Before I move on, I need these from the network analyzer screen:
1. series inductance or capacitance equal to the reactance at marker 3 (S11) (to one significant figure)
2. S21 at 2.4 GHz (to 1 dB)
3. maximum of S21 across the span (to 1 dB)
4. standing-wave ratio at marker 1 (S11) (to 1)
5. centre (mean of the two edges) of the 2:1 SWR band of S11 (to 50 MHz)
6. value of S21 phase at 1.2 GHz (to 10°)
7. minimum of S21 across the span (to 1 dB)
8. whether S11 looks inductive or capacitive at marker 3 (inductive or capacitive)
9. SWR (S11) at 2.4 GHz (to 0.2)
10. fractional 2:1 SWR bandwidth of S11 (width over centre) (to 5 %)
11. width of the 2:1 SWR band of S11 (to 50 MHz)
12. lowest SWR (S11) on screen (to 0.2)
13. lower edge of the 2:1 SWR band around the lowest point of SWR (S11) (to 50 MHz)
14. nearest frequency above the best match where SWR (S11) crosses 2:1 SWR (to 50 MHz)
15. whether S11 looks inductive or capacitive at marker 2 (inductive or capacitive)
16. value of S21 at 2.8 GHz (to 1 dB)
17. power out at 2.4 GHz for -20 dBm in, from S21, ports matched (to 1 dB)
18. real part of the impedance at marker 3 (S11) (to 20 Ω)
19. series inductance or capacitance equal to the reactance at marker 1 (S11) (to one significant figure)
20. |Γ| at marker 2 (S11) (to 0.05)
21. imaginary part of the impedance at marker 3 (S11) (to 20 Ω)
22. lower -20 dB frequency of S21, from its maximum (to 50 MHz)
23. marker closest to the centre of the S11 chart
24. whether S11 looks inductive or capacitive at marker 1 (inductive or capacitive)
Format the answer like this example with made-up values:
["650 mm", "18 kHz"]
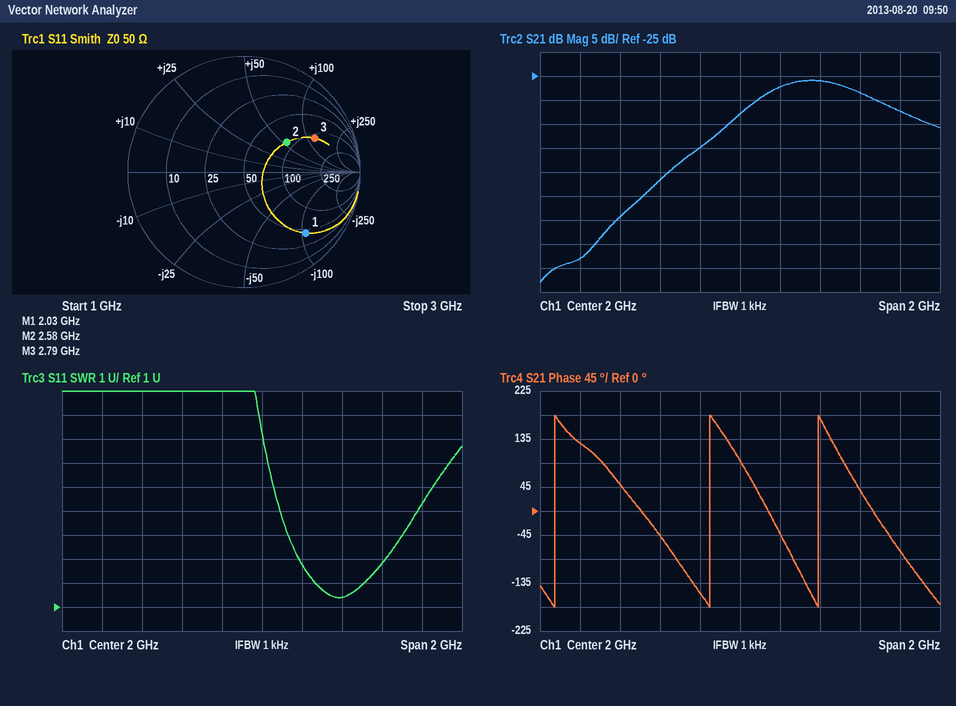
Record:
["7 nH", "-26 dB", "-26 dB", "7", "2.40 GHz", "130°", "-68 dB", "inductive", "1.4", "10 %", "250 MHz", "1.4", "2.25 GHz", "2.50 GHz", "inductive", "-32 dB", "-46 dBm", "120 Ω", "700 fF", "0.45", "+120 Ω", "1.60 GHz", "marker 2", "capacitive"]
